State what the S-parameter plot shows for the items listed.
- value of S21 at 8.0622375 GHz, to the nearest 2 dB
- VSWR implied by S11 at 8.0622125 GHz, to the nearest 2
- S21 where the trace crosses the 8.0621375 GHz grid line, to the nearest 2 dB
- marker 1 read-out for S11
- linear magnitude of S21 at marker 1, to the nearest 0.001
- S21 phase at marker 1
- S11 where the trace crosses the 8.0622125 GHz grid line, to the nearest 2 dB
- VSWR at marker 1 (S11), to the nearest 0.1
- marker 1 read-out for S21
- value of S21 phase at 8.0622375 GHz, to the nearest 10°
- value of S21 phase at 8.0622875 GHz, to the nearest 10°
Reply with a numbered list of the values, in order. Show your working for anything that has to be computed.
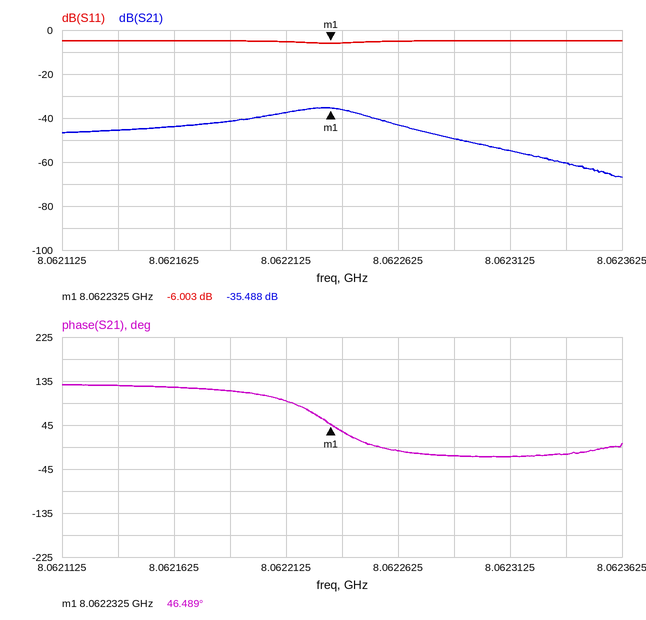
1. -36 dB
2. |Γ| = 10^(-6/20) = 0.5012; VSWR = (1 + 0.5012)/(1 − 0.5012) ≈ 3.01, so 4 to the nearest 2
3. -46 dB
4. -6.003 dB
5. 10^(-35.488/20) ≈ 0.017
6. 46.489°
7. -6 dB
8. (1 + 0.5010)/(1 − 0.5010) ≈ 3.0
9. -35.488 dB
10. 30°
11. -20°
